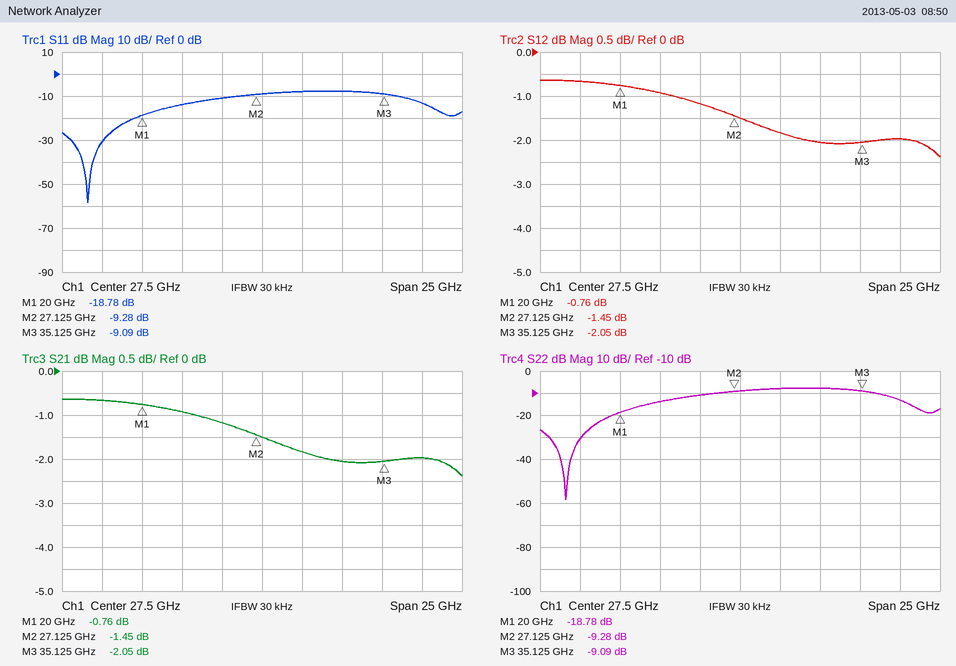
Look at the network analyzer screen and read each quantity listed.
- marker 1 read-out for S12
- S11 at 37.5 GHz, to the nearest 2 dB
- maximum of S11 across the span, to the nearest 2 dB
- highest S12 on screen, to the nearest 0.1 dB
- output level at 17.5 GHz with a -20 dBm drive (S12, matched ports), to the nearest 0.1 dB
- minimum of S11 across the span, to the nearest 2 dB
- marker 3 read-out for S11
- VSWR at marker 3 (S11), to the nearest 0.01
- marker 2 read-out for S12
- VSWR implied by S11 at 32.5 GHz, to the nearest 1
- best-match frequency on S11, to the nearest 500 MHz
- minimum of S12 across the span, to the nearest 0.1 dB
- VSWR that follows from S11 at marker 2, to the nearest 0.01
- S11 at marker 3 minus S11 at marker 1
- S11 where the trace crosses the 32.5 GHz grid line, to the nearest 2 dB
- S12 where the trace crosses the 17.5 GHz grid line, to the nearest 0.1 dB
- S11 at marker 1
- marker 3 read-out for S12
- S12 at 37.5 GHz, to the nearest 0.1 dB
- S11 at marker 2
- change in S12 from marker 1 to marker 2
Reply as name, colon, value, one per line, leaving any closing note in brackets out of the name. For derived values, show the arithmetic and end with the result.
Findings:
marker 1 read-out for S12: -0.76 dB
S11 at 37.5 GHz, to the nearest 2 dB: -14 dB
maximum of S11 across the span, to the nearest 2 dB: -8 dB
highest S12 on screen, to the nearest 0.1 dB: -0.6 dB
output level at 17.5 GHz with a -20 dBm drive (S12, matched ports), to the nearest 0.1 dB: -20 dBm + (-0.7 dB) = -20.7 dBm
minimum of S11 across the span, to the nearest 2 dB: -58 dB
marker 3 read-out for S11: -9.09 dB
VSWR at marker 3 (S11), to the nearest 0.01: (1 + 0.3512)/(1 − 0.3512) ≈ 2.08
marker 2 read-out for S12: -1.45 dB
VSWR implied by S11 at 32.5 GHz, to the nearest 1: |Γ| = 10^(-8/20) = 0.3981; VSWR = (1 + 0.3981)/(1 − 0.3981) ≈ 2
best-match frequency on S11, to the nearest 500 MHz: 16.5 GHz
minimum of S12 across the span, to the nearest 0.1 dB: -2.4 dB
VSWR that follows from S11 at marker 2, to the nearest 0.01: (1 + 0.3436)/(1 − 0.3436) ≈ 2.05
S11 at marker 3 minus S11 at marker 1: -9.09 − (-18.78) = 9.69 dB
S11 where the trace crosses the 32.5 GHz grid line, to the nearest 2 dB: -8 dB
S12 where the trace crosses the 17.5 GHz grid line, to the nearest 0.1 dB: -0.7 dB
S11 at marker 1: -18.78 dB
marker 3 read-out for S12: -2.05 dB
S12 at 37.5 GHz, to the nearest 0.1 dB: -2.0 dB
S11 at marker 2: -9.28 dB
change in S12 from marker 1 to marker 2: -1.45 − (-0.76) = -0.69 dB
